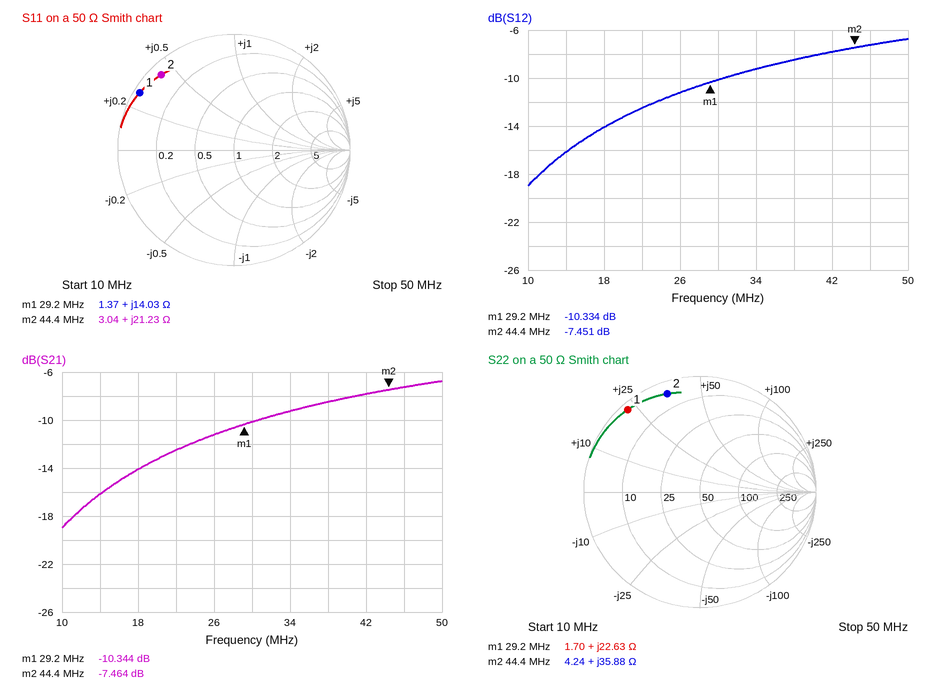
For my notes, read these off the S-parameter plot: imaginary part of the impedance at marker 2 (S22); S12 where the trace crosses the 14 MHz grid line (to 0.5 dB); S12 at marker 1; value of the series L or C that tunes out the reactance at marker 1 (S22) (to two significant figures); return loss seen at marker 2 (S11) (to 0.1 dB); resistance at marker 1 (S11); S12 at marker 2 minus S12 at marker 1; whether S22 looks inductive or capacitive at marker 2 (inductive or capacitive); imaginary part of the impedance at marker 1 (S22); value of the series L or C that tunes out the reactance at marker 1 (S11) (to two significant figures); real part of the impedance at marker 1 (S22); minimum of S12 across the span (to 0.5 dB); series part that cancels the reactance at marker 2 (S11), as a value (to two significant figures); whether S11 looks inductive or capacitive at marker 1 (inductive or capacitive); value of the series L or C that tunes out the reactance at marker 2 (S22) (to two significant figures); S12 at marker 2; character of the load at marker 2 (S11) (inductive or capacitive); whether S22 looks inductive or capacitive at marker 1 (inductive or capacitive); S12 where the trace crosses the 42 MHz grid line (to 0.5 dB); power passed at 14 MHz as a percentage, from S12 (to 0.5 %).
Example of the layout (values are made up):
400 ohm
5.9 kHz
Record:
+35.88 Ω
-16.0 dB
-10.334 dB
240 pF
0.9 dB
1.37 Ω
2.883 dB
inductive
+22.63 Ω
390 pF
1.70 Ω
-19.0 dB
170 pF
inductive
100 pF
-7.451 dB
inductive
inductive
-8.0 dB
2.5 %
